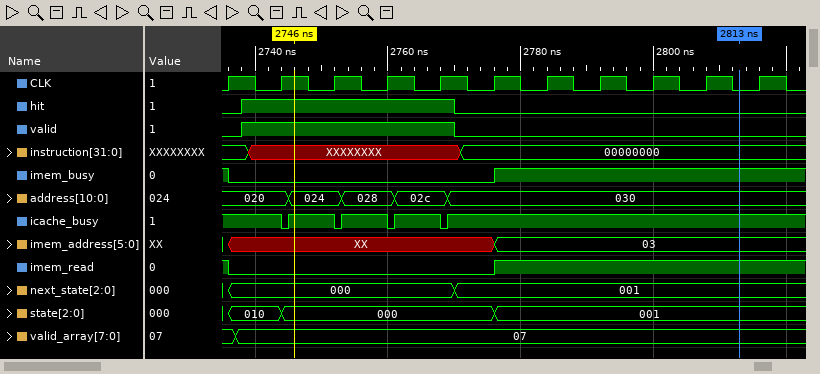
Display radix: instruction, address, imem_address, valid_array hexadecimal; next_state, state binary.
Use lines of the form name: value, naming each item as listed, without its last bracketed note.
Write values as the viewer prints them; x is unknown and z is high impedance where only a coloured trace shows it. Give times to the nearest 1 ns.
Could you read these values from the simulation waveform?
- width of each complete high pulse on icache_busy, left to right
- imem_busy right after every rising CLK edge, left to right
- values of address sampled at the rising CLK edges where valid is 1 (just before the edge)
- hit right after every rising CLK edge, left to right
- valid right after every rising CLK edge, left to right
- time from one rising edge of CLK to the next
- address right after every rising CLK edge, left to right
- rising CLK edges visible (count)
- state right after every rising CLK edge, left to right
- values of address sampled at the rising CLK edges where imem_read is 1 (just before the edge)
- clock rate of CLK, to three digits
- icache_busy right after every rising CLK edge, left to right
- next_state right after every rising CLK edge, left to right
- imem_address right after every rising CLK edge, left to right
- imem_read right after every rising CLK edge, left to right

width of each complete high pulse on icache_busy, left to right: 7 ns, 7 ns, 7 ns
imem_busy right after every rising CLK edge, left to right: 0 0 0 0 0 1 1 1 1 1 1
values of address sampled at the rising CLK edges where valid is 1: 020, 024, 028, 02c
hit right after every rising CLK edge, left to right: 0 1 1 1 1 0 0 0 0 0 0
valid right after every rising CLK edge, left to right: 0 1 1 1 1 0 0 0 0 0 0
time from one rising edge of CLK to the next: 8 ns
address right after every rising CLK edge, left to right: 020, 020, 024, 028, 02c, 030, 030, 030, 030, 030, 030
rising CLK edges visible: 11
state right after every rising CLK edge, left to right: 010, 000, 000, 000, 000, 001, 001, 001, 001, 001, 001
values of address sampled at the rising CLK edges where imem_read is 1: 020, 030, 030, 030, 030, 030
clock rate of CLK, to three digits: 125 MHz
icache_busy right after every rising CLK edge, left to right: 1 0 0 0 0 1 1 1 1 1 1
next_state right after every rising CLK edge, left to right: 000, 000, 000, 000, 000, 001, 001, 001, 001, 001, 001
imem_address right after every rising CLK edge, left to right: XX, XX, XX, XX, XX, 03, 03, 03, 03, 03, 03
imem_read right after every rising CLK edge, left to right: 0 0 0 0 0 1 1 1 1 1 1
